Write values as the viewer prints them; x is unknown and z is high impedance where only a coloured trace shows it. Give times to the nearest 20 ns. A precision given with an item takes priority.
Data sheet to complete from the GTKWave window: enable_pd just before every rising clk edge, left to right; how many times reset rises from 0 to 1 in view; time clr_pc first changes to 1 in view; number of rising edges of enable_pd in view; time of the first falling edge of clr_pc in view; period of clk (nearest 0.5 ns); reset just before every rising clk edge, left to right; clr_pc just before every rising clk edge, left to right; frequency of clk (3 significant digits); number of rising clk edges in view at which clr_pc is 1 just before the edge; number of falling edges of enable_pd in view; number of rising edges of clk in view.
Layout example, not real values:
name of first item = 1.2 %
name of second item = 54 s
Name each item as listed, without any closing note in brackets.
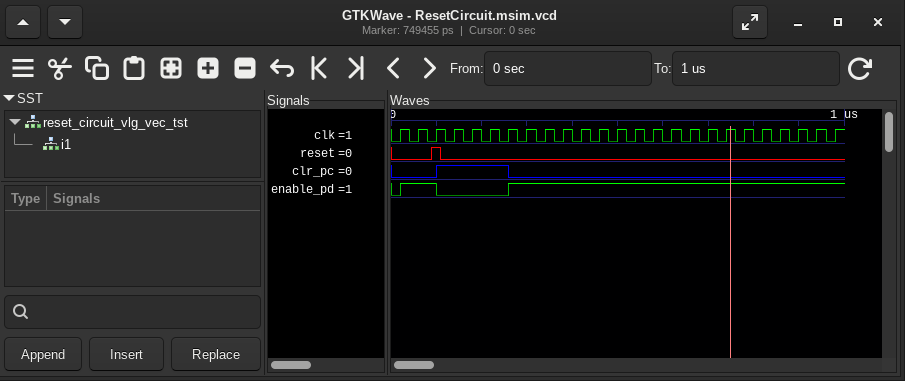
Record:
enable_pd just before every rising clk edge, left to right = 0 1 1 0 0 0 0 1 1 1 1 1 1 1 1 1 1 1 1 1 1 1 1 1 1
how many times reset rises from 0 to 1 in view = 1
time clr_pc first changes to 1 in view = 100 ns
number of rising edges of enable_pd in view = 2
time of the first falling edge of clr_pc in view = 260 ns
period of clk = 40 ns
reset just before every rising clk edge, left to right = 0 0 1 0 0 0 0 0 0 0 0 0 0 0 0 0 0 0 0 0 0 0 0 0 0
clr_pc just before every rising clk edge, left to right = 0 0 0 1 1 1 1 0 0 0 0 0 0 0 0 0 0 0 0 0 0 0 0 0 0
frequency of clk = 25.0 MHz
number of rising clk edges in view at which clr_pc is 1 just before the edge = 4
number of falling edges of enable_pd in view = 1
number of rising edges of clk in view = 25
